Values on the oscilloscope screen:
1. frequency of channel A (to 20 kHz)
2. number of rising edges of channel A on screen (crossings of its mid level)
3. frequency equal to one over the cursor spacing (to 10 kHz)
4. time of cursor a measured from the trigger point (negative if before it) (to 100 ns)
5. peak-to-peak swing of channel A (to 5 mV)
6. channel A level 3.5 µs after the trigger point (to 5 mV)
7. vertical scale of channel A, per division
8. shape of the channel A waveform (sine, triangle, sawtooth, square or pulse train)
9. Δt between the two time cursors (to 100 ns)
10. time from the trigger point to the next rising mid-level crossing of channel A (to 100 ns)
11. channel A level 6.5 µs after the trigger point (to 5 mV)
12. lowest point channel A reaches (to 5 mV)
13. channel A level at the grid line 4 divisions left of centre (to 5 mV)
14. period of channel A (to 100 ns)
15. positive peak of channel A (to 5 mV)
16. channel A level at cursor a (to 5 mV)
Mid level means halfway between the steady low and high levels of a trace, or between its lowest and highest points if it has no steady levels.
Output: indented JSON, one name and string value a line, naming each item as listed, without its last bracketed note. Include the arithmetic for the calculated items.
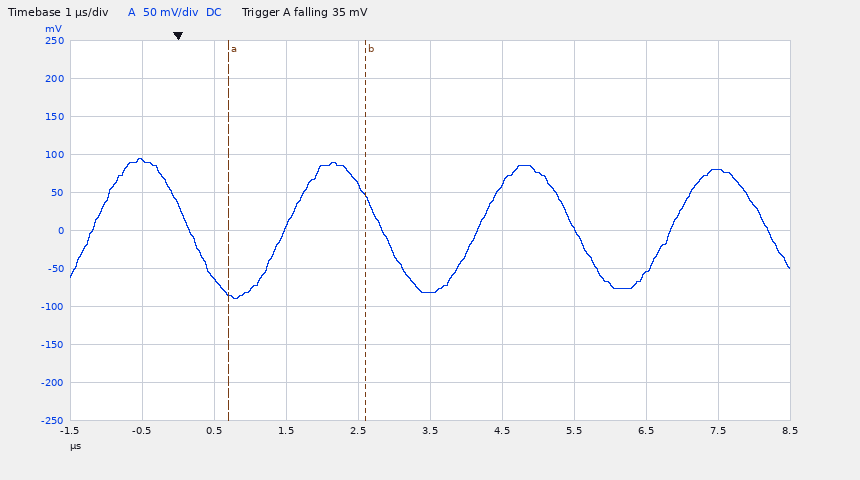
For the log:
{
  "frequency of channel A": "1 / 2.7 µs ≈ 370 kHz, so 380 kHz to the nearest 20 kHz",
  "number of rising edges of channel A on screen": "4",
  "frequency equal to one over the cursor spacing": "1 / 1.9 µs ≈ 530 kHz",
  "time of cursor a measured from the trigger point (negative if before it)": "+700 ns",
  "peak-to-peak swing of channel A": "95 mV − (-90 mV) = 185 mV",
  "channel A level 3.5 µs after the trigger point": "-80 mV",
  "vertical scale of channel A, per division": "50 mV",
  "shape of the channel A waveform": "sine",
  "Δt between the two time cursors": "1.9 µs",
  "time from the trigger point to the next rising mid-level crossing of channel A": "1.5 µs",
  "channel A level 6.5 µs after the trigger point": "-55 mV",
  "lowest point channel A reaches": "-90 mV",
  "channel A level at the grid line 4 divisions left of centre": "90 mV",
  "period of channel A": "2.7 µs",
  "positive peak of channel A": "95 mV",
  "channel A level at cursor a": "-85 mV"
}
